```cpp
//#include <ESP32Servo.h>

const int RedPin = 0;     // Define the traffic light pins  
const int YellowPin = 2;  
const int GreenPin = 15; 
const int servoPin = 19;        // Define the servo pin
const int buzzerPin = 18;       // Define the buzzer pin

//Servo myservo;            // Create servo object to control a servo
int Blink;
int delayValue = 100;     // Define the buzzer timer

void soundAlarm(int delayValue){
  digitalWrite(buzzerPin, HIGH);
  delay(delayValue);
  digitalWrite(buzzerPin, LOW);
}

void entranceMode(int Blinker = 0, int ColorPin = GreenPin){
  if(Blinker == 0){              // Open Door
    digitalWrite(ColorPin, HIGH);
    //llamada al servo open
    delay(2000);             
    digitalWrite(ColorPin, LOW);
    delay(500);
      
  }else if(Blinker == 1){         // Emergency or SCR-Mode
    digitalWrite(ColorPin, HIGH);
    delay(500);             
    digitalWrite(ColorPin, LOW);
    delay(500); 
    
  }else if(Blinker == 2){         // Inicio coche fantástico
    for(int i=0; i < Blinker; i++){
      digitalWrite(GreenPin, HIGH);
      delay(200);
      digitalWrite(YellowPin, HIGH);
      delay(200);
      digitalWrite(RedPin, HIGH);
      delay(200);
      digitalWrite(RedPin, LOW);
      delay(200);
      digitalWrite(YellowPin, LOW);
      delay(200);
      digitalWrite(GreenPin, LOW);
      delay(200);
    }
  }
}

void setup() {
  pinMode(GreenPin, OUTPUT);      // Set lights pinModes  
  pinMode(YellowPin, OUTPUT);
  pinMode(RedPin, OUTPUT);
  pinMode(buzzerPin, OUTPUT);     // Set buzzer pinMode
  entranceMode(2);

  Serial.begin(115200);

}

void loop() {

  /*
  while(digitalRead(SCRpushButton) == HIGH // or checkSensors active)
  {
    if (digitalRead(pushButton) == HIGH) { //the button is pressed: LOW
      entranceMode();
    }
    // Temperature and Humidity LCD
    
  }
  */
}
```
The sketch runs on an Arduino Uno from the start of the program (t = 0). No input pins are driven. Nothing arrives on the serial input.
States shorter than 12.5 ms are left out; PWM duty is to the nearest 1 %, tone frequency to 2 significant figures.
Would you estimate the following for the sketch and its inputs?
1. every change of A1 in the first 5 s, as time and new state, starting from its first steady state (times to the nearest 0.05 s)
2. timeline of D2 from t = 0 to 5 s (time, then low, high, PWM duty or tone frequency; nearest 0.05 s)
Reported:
0 s high; 1 s low; 1.2 s high; 2.2 s low
0 s low; 0.2 s high; 0.8 s low; 1.4 s high; 2 s low
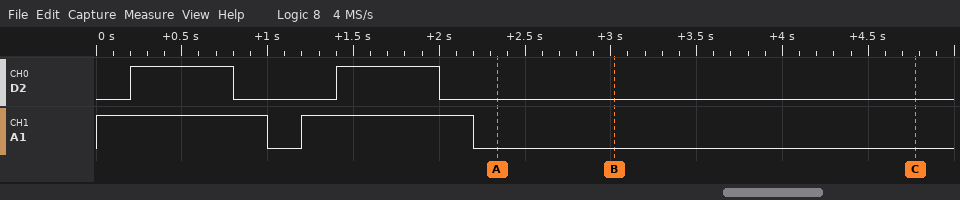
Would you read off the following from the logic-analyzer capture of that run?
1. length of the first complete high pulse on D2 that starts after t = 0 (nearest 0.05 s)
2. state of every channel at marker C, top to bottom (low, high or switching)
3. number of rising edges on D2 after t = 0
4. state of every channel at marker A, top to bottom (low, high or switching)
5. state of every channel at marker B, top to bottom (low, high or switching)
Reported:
0.60 s
D2 low, A1 low
2
D2 low, A1 low
D2 low, A1 low
